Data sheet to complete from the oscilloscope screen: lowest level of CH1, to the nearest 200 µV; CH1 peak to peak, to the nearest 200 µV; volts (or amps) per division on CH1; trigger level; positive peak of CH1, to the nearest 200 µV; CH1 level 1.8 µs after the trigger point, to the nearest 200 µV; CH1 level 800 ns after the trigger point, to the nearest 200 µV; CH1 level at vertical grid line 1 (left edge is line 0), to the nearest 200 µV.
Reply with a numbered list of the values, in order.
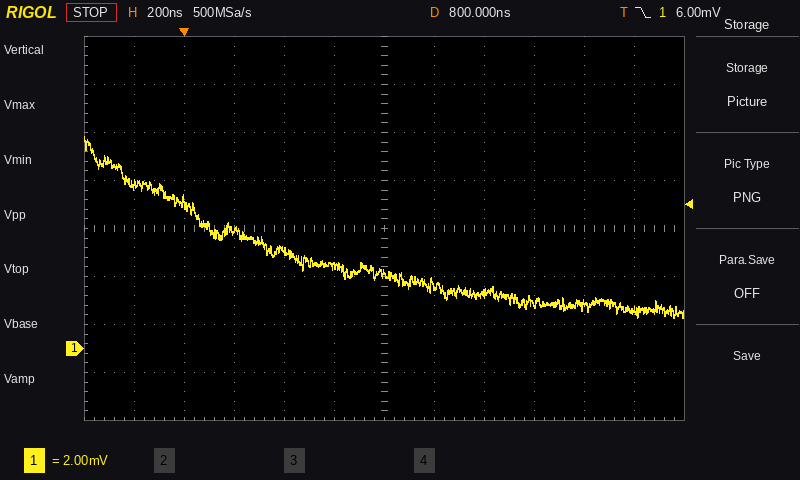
1. 1.2 mV
2. 7.6 mV
3. 2 mV
4. 6.00 mV
5. 8.8 mV
6. 1.6 mV
7. 3.2 mV
8. 6.8 mV
